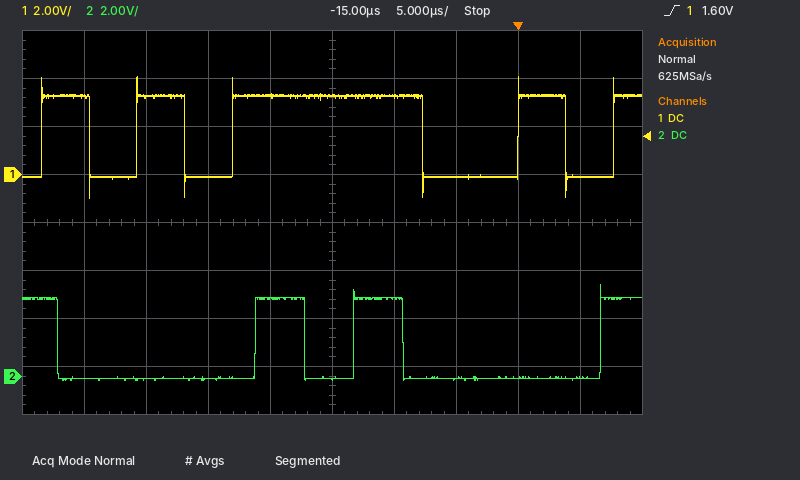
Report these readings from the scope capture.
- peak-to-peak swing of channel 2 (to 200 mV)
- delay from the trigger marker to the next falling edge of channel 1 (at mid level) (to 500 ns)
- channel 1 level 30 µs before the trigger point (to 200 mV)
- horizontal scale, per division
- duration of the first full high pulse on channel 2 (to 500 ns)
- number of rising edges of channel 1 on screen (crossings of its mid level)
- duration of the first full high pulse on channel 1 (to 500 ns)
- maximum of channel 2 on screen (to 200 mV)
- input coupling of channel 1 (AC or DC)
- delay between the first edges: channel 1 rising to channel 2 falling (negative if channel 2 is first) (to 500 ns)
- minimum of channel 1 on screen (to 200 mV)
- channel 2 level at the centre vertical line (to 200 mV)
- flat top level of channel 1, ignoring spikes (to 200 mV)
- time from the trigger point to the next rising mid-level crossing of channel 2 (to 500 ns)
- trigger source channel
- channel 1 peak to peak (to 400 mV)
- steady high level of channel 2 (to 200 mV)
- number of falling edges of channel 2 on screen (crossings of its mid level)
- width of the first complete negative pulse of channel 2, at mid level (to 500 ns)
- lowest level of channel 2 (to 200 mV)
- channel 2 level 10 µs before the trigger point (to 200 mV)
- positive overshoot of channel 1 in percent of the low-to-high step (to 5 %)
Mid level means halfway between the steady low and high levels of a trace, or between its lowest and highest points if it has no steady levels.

4.0 V
4.0 µs
3.2 V
5 µs
4.0 µs
5
4.0 µs
3.8 V
DC
+1.5 µs
-1.0 V
-200 mV
3.2 V
6.5 µs
channel 1
5.2 V
3.2 V
3
16.0 µs
-200 mV
3.2 V
25 %
